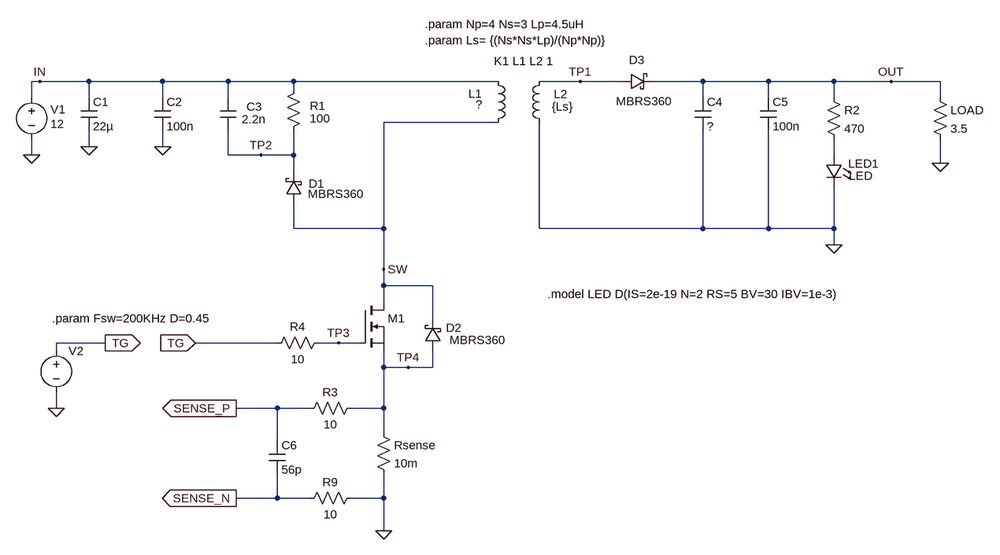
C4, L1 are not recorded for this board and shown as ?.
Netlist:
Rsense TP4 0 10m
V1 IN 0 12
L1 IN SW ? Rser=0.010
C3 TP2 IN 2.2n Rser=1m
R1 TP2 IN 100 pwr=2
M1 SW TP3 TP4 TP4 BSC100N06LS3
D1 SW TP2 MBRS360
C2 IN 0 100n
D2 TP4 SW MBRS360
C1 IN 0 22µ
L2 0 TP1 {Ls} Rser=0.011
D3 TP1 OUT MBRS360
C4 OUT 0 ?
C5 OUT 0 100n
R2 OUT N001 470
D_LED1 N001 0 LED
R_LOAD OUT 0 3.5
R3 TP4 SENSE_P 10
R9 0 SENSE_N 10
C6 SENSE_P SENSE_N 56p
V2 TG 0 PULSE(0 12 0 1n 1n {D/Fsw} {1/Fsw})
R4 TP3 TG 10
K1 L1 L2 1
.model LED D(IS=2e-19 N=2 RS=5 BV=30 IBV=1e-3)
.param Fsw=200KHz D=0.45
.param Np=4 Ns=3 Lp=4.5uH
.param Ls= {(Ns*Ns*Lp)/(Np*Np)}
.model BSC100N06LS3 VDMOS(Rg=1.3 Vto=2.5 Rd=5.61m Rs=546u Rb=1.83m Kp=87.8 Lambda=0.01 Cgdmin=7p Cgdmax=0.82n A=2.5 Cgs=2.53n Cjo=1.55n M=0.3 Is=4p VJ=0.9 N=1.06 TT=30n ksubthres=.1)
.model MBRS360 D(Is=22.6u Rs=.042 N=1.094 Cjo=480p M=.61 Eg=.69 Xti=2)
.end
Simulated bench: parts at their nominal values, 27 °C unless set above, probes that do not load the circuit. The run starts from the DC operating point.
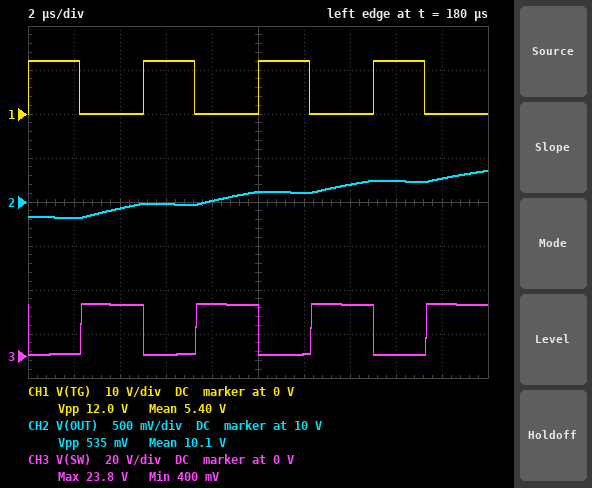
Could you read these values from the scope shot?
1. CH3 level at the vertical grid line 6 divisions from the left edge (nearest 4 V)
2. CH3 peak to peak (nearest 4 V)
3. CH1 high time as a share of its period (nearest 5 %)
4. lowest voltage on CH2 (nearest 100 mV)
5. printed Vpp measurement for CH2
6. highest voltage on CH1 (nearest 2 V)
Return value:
0 V
24 V
45 %
9.8 V
535 mV
12 V
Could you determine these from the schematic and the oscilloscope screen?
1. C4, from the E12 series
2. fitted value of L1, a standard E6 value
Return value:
560 µF
2.2 µH
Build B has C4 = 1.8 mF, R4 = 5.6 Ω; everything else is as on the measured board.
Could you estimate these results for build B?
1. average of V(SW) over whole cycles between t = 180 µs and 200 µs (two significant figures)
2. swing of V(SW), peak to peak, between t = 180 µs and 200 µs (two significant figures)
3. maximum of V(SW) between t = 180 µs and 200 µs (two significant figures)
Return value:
12 V
20 V
21 V
